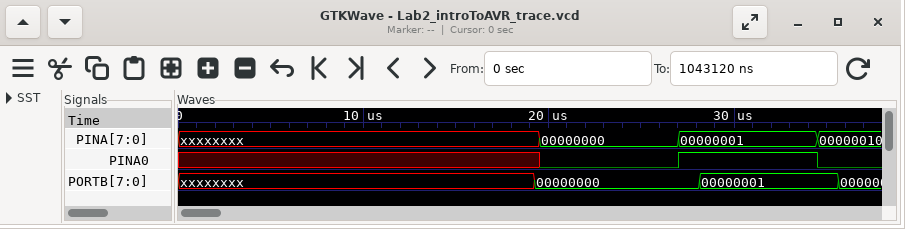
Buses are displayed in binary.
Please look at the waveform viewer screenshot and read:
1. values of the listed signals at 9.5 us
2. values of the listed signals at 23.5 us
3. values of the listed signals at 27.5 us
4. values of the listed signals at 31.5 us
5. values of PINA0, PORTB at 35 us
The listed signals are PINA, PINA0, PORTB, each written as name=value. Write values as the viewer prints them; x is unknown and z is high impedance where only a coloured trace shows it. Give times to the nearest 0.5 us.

PINA=xxxxxxxx, PINA0=x, PORTB=xxxxxxxx
PINA=00000000, PINA0=0, PORTB=00000000
PINA=00000001, PINA0=1, PORTB=00000000
PINA=00000001, PINA0=1, PORTB=00000001
PINA0=0, PORTB=00000001
